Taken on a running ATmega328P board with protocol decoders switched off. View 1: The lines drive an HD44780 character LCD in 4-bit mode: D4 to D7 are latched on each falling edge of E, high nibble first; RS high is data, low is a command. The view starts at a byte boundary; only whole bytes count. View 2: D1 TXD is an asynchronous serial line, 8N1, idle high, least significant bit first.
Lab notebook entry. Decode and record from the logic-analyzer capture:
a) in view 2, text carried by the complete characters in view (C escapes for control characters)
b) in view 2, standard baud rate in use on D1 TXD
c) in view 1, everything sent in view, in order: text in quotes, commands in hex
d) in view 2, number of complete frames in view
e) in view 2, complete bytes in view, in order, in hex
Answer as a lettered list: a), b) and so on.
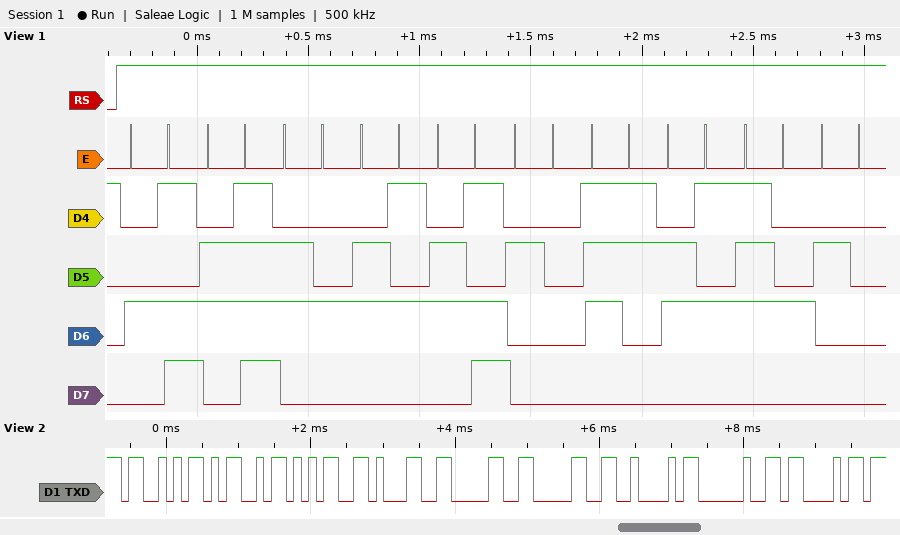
a) "SM5100B C"
b) 9600 baud
c) "Modem set "
d) 9
e) 0x53 0x4D 0x35 0x31 0x30 0x30 0x42 0x20 0x43
